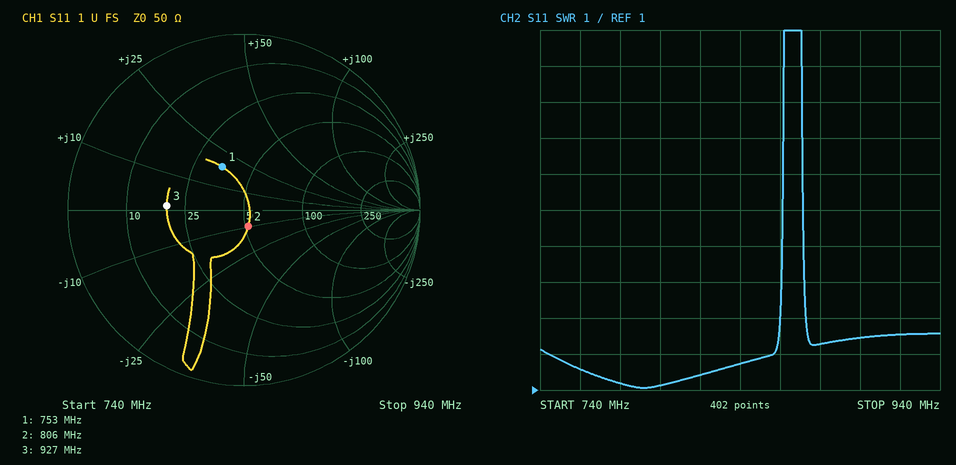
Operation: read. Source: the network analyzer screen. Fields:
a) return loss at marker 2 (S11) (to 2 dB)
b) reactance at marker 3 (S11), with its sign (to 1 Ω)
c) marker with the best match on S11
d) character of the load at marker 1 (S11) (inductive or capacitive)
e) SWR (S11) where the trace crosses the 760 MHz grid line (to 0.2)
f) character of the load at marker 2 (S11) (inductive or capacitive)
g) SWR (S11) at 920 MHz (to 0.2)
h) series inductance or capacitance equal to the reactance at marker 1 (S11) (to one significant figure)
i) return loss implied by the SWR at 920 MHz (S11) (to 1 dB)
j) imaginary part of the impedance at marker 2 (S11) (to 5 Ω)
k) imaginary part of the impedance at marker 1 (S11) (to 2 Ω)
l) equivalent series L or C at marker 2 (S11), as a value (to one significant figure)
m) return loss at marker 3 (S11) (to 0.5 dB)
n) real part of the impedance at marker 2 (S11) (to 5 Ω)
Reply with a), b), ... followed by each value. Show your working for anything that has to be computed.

a) 20 dB
b) +1 Ω
c) marker 2
d) inductive
e) 1.6
f) capacitive
g) 2.6
h) L = 18 Ω/(2π × 753 MHz) ≈ 4 nH
i) −20 log10((2.6 − 1)/(2.6 + 1)) ≈ 7 dB
j) -10 Ω
k) +18 Ω
l) C = 1/(2π × 806 MHz × 10 Ω) ≈ 20 pF
m) 7.0 dB
n) 50 Ω
